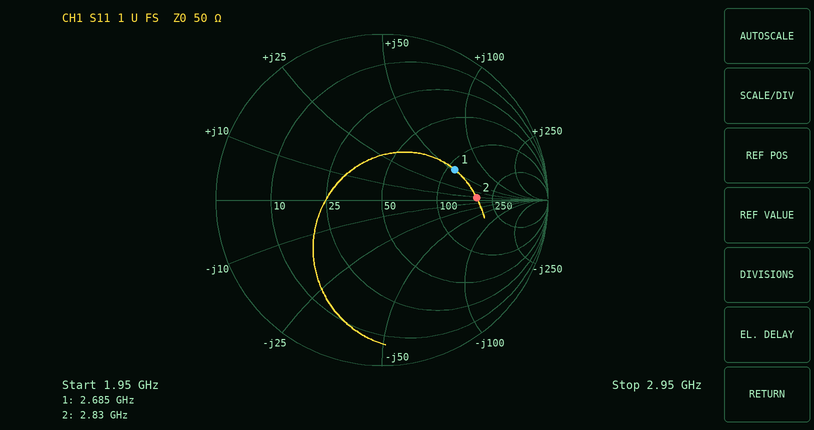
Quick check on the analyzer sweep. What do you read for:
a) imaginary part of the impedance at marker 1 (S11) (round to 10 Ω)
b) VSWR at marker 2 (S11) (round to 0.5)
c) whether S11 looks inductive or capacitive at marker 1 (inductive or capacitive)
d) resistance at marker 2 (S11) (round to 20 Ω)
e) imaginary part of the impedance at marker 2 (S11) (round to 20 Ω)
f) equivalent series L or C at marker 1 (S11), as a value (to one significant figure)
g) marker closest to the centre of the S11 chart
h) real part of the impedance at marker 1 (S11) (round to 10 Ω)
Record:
+50 Ω
3.5
inductive
180 Ω
0 Ω
3 nH
marker 1
110 Ω
